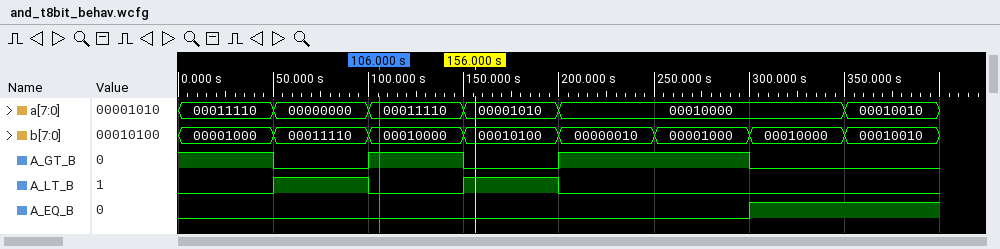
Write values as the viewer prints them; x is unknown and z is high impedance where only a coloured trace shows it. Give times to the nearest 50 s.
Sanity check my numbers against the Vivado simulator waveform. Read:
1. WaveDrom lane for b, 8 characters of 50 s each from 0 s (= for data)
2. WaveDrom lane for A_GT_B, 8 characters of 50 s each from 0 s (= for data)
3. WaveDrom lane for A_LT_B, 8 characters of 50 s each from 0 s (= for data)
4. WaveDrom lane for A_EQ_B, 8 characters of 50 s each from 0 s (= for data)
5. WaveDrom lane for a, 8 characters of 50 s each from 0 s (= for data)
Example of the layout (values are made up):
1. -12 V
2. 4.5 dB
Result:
1. {name: 'b', wave: '========', data: '00001000 00011110 00010000 00010100 00000010 00001000 00010000 00010010'}
2. {name: 'A_GT_B', wave: '10101.0.'}
3. {name: 'A_LT_B', wave: '01010...'}
4. {name: 'A_EQ_B', wave: '0.....1.'}
5. {name: 'a', wave: '=====..=', data: '00011110 00000000 00011110 00001010 00010000 00010010'}
